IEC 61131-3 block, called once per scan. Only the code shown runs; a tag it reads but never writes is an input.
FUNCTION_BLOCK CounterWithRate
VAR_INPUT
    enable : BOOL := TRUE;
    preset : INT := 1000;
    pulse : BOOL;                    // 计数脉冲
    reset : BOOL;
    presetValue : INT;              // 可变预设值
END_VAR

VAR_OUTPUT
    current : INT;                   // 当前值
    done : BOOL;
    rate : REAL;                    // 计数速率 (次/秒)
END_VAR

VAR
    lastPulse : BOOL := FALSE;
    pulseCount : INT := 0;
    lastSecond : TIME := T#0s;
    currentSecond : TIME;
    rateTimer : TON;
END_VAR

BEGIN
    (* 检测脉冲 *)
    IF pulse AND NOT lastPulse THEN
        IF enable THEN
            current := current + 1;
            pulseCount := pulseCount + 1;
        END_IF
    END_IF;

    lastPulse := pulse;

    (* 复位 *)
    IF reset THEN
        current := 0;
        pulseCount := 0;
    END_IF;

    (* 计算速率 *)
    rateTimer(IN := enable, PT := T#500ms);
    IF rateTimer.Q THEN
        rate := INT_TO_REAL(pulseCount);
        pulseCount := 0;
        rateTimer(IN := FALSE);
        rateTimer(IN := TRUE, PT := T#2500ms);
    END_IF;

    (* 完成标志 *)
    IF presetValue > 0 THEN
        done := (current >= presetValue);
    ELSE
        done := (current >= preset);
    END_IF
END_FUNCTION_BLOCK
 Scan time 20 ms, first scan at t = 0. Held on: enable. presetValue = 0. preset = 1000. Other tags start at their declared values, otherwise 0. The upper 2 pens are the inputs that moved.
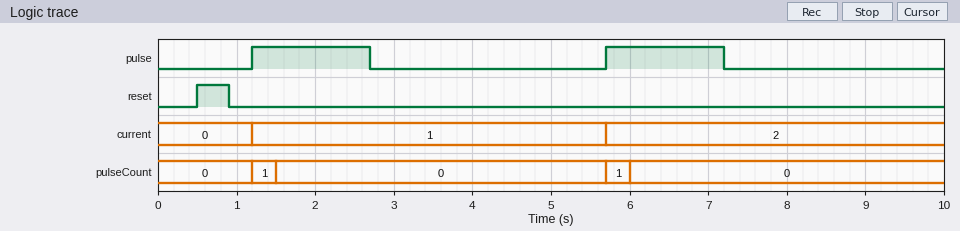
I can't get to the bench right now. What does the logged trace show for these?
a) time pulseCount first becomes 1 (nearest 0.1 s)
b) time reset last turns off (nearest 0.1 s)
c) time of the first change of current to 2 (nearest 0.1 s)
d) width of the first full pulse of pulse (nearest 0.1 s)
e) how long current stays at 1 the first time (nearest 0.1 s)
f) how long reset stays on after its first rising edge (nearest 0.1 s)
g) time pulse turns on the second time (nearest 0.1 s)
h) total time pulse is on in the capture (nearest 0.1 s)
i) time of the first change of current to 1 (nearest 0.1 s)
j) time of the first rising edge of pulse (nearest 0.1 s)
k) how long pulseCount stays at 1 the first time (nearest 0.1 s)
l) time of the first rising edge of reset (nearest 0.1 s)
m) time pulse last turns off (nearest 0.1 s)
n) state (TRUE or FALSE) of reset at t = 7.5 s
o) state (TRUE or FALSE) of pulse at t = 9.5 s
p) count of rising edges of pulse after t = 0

1.2 s
0.9 s
5.7 s
1.5 s
4.5 s
0.4 s
5.7 s
3.0 s
1.2 s
1.2 s
0.3 s
0.5 s
7.2 s
FALSE
FALSE
2
